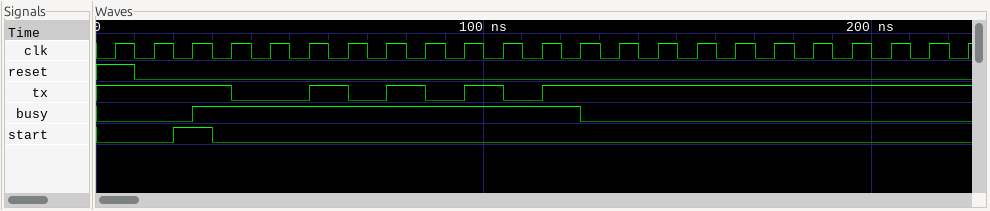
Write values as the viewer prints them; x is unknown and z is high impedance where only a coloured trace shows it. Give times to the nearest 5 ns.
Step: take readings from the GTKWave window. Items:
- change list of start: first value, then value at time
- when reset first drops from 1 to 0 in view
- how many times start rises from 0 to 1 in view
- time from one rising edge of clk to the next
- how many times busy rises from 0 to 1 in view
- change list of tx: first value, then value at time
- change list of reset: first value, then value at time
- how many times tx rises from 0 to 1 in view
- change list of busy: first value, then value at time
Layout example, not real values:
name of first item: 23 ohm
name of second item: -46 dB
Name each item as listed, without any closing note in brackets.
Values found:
change list of start: first value, then value at time: 0, 1 at 20 ns, 0 at 30 ns
when reset first drops from 1 to 0 in view: 10 ns
how many times start rises from 0 to 1 in view: 1
time from one rising edge of clk to the next: 10 ns
how many times busy rises from 0 to 1 in view: 1
change list of tx: first value, then value at time: 1, 0 at 35 ns, 1 at 55 ns, 0 at 65 ns, 1 at 75 ns, 0 at 85 ns, 1 at 95 ns, 0 at 105 ns, 1 at 115 ns
change list of reset: first value, then value at time: 1, 0 at 10 ns
how many times tx rises from 0 to 1 in view: 4
change list of busy: first value, then value at time: 0, 1 at 25 ns, 0 at 125 ns
